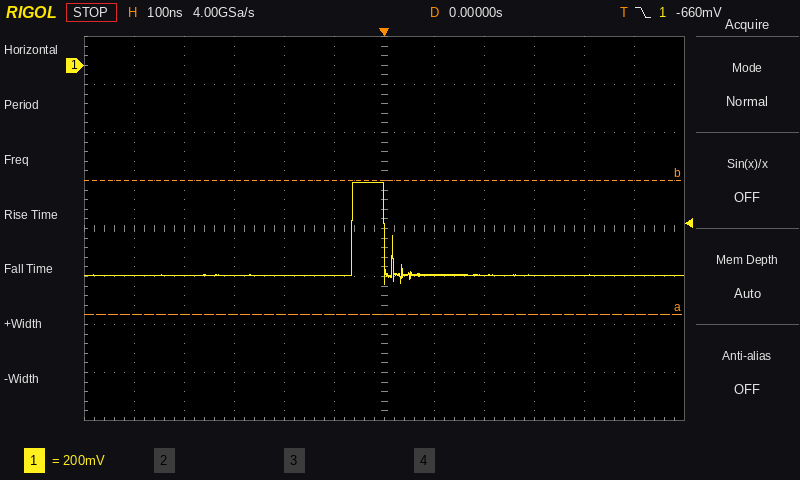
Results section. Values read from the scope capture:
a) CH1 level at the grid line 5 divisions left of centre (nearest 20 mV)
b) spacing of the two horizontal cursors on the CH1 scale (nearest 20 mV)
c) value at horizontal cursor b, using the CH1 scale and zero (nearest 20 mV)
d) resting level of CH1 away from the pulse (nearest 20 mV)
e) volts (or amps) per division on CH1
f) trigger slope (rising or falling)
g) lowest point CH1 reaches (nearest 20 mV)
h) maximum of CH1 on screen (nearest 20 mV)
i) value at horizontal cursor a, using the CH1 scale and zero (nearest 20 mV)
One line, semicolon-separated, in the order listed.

-880 mV; 560 mV; -480 mV; -880 mV; 200 mV; falling; -920 mV; -480 mV; -1.04 V
